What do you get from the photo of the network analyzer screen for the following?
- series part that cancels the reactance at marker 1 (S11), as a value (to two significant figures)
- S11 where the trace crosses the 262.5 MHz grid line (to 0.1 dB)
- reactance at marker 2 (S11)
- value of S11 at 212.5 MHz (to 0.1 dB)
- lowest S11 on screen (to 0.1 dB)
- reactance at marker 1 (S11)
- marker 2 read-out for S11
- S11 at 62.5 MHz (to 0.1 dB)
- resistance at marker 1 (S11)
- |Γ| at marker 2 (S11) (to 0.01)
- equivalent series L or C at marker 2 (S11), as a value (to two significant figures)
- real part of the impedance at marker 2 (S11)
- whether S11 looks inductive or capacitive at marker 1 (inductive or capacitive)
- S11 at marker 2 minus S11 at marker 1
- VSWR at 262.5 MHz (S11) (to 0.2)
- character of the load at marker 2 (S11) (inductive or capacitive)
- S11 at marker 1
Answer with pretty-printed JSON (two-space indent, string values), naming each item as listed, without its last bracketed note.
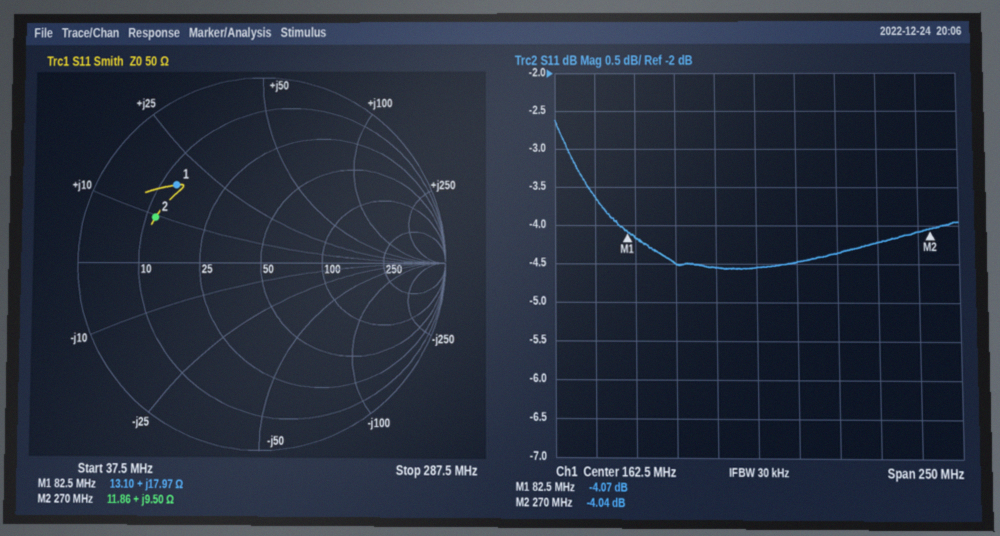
{
  "series part that cancels the reactance at marker 1 (S11), as a value": "110 pF",
  "S11 where the trace crosses the 262.5 MHz grid line": "-4.1 dB",
  "reactance at marker 2": "+9.50 Ω",
  "value of S11 at 212.5 MHz": "-4.4 dB",
  "lowest S11 on screen": "-4.6 dB",
  "reactance at marker 1": "+17.97 Ω",
  "marker 2 read-out for S11": "-4.04 dB",
  "S11 at 62.5 MHz": "-3.6 dB",
  "resistance at marker 1": "13.10 Ω",
  "|Γ| at marker 2 (S11)": "0.63",
  "equivalent series L or C at marker 2 (S11), as a value": "5.6 nH",
  "real part of the impedance at marker 2": "11.86 Ω",
  "whether S11 looks inductive or capacitive at marker 1": "inductive",
  "S11 at marker 2 minus S11 at marker 1": "0.03 dB",
  "VSWR at 262.5 MHz (S11)": "4.4",
  "character of the load at marker 2 (S11)": "inductive",
  "S11 at marker 1": "-4.07 dB"
}
